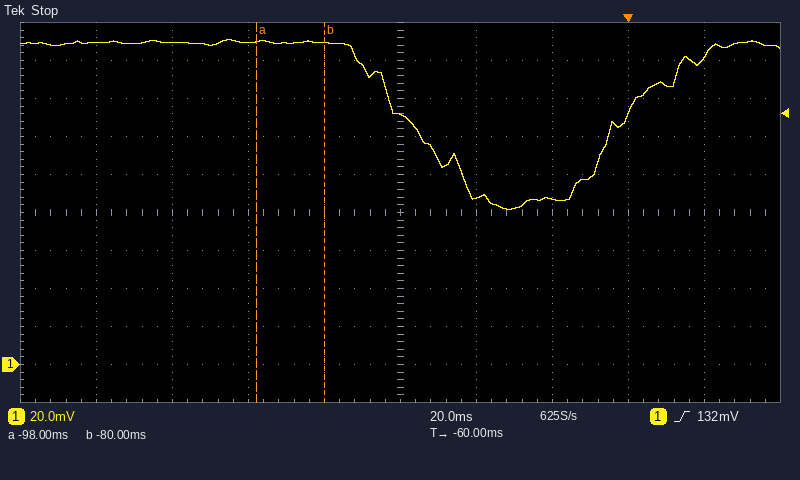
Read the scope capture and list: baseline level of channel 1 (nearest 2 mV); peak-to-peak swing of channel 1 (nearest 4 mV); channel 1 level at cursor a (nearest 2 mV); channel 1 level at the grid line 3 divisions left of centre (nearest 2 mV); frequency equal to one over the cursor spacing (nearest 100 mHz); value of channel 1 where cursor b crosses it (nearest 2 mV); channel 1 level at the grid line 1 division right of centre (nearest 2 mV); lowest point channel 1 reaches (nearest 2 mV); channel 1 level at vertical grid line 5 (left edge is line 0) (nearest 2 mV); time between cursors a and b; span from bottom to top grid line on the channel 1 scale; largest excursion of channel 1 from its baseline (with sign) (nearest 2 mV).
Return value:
170 mV
88 mV
170 mV
170 mV
55.6 Hz
170 mV
88 mV
82 mV
132 mV
18 ms
200 mV
-88 mV
